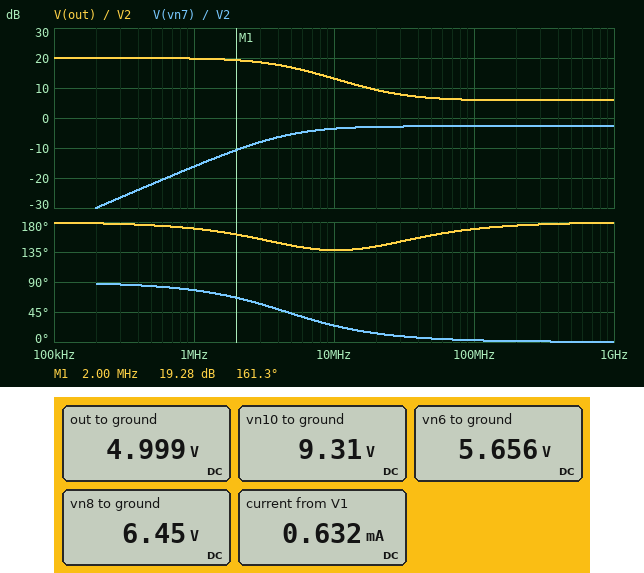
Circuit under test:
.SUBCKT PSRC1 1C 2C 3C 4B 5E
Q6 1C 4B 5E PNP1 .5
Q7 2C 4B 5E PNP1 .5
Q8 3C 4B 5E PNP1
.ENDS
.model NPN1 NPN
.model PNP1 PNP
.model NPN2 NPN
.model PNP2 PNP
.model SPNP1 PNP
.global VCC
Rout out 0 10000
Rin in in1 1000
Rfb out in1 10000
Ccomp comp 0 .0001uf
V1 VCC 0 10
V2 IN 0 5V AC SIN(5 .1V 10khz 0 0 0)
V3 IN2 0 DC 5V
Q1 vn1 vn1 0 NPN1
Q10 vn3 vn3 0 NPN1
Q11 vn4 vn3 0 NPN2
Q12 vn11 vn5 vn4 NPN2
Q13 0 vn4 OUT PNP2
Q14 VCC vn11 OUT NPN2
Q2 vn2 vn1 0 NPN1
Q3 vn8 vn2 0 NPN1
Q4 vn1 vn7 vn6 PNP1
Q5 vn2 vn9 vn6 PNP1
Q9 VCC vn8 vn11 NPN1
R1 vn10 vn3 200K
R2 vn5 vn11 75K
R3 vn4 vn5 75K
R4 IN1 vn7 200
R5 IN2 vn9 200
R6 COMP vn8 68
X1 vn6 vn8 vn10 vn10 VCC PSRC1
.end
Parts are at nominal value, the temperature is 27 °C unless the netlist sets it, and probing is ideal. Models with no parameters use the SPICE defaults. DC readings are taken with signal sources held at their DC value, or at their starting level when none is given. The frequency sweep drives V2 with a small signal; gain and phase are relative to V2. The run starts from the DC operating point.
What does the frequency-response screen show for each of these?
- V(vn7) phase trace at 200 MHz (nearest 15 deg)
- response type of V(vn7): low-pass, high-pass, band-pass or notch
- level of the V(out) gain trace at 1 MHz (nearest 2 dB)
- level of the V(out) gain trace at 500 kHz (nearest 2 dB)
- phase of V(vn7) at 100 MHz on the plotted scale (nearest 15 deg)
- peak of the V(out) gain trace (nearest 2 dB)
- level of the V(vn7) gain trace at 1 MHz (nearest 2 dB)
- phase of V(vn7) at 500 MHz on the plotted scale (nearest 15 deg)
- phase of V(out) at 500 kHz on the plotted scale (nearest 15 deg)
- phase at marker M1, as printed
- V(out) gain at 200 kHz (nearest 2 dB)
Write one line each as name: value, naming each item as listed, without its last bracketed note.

V(vn7) phase trace at 200 MHz: 0 deg
response type of V(vn7): low-pass, high-pass, band-pass or notch: high-pass
level of the V(out) gain trace at 1 MHz: 20 dB
level of the V(out) gain trace at 500 kHz: 20 dB
phase of V(vn7) at 100 MHz on the plotted scale: 0 deg
peak of the V(out) gain trace: 20 dB
level of the V(vn7) gain trace at 1 MHz: -16 dB
phase of V(vn7) at 500 MHz on the plotted scale: 0 deg
phase of V(out) at 500 kHz on the plotted scale: 180 deg
phase at marker M1, as printed: 161.3 deg
V(out) gain at 200 kHz: 20 dB
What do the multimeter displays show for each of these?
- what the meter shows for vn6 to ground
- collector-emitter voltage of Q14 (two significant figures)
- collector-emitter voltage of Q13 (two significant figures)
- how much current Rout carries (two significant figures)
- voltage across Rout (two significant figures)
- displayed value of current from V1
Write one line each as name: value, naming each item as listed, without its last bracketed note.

what the meter shows for vn6 to ground: 5.656 V
collector-emitter voltage of Q14: 5.0 V
collector-emitter voltage of Q13: -5.0 V
how much current Rout carries: 500 µA
voltage across Rout: 5.0 V
displayed value of current from V1: 0.632 mA
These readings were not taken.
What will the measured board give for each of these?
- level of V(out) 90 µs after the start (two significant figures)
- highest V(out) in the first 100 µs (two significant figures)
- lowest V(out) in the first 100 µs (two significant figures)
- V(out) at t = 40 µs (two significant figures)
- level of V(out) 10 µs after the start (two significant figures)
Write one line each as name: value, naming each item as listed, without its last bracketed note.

level of V(out) 90 µs after the start: 5.6 V
highest V(out) in the first 100 µs: 6.0 V
lowest V(out) in the first 100 µs: 4.0 V
V(out) at t = 40 µs: 4.4 V
level of V(out) 10 µs after the start: 4.4 V
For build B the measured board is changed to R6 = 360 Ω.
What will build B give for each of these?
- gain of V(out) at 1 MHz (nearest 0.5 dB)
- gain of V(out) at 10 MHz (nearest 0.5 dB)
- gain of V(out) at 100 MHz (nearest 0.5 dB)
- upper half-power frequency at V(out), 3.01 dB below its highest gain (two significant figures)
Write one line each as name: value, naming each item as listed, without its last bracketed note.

gain of V(out) at 1 MHz: 19.5 dB
gain of V(out) at 10 MHz: 15.5 dB
gain of V(out) at 100 MHz: 15.0 dB
upper half-power frequency at V(out), 3.01 dB below its highest gain: 4.1 MHz
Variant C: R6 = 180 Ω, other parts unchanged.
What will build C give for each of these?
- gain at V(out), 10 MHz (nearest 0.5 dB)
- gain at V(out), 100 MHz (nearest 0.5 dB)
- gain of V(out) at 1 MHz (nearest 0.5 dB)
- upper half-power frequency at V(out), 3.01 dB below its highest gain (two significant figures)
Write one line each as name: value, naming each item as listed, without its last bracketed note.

gain at V(out), 10 MHz: 14.0 dB
gain at V(out), 100 MHz: 12.0 dB
gain of V(out) at 1 MHz: 19.5 dB
upper half-power frequency at V(out), 3.01 dB below its highest gain: 4.2 MHz
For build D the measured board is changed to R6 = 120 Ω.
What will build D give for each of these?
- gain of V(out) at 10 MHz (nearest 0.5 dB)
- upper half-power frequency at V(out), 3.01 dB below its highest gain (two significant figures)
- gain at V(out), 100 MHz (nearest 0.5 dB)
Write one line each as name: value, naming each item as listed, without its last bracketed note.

gain of V(out) at 10 MHz: 13.5 dB
upper half-power frequency at V(out), 3.01 dB below its highest gain: 4.4 MHz
gain at V(out), 100 MHz: 9.5 dB
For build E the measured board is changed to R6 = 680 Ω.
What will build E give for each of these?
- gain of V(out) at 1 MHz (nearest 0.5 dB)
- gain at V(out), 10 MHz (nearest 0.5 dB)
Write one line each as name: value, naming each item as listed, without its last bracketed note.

gain of V(out) at 1 MHz: 19.5 dB
gain at V(out), 10 MHz: 17.0 dB
